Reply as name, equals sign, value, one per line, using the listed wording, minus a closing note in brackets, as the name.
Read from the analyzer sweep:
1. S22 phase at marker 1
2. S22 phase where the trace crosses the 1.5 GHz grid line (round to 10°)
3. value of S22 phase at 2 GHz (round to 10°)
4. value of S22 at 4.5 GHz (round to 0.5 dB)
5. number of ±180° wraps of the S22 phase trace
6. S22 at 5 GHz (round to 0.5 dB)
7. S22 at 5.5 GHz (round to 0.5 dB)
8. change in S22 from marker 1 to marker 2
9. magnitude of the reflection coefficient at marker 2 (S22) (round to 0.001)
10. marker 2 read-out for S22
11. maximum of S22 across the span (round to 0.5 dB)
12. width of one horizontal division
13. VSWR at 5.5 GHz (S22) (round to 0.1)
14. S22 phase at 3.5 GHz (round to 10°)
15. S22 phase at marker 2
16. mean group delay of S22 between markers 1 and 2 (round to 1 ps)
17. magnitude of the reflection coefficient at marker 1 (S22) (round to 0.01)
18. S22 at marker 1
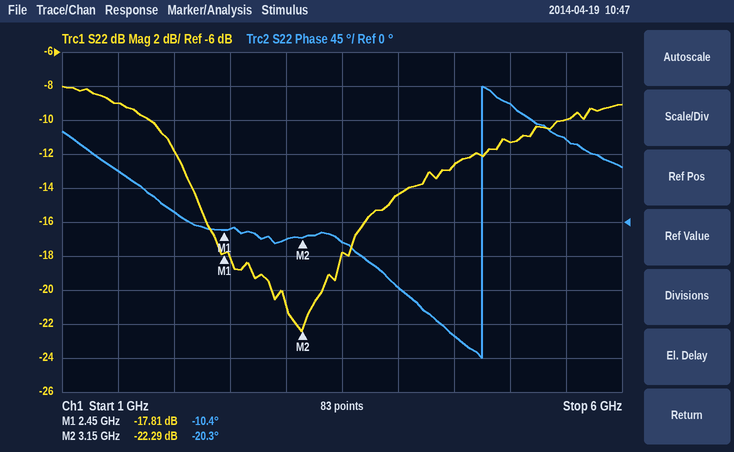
S22 phase at marker 1 = -10.4°
S22 phase where the trace crosses the 1.5 GHz grid line = 70°
value of S22 phase at 2 GHz = 10°
value of S22 at 4.5 GHz = -12.5 dB
number of ±180° wraps of the S22 phase trace = 1
S22 at 5 GHz = -11.5 dB
S22 at 5.5 GHz = -10.0 dB
change in S22 from marker 1 to marker 2 = -4.48 dB
magnitude of the reflection coefficient at marker 2 (S22) = 0.077
marker 2 read-out for S22 = -22.29 dB
maximum of S22 across the span = -8.0 dB
width of one horizontal division = 500 MHz
VSWR at 5.5 GHz (S22) = 1.9
S22 phase at 3.5 GHz = -30°
S22 phase at marker 2 = -20.3°
mean group delay of S22 between markers 1 and 2 = 39 ps
magnitude of the reflection coefficient at marker 1 (S22) = 0.13
S22 at marker 1 = -17.81 dB
